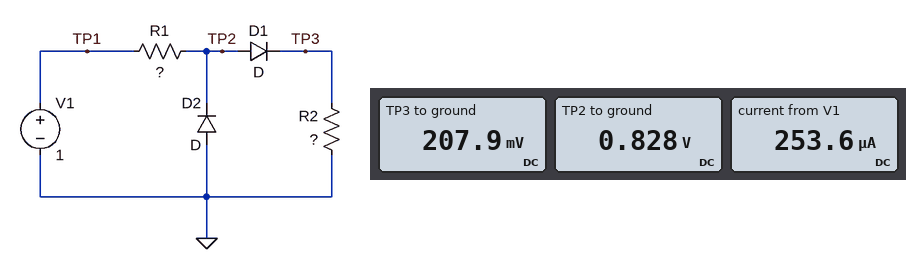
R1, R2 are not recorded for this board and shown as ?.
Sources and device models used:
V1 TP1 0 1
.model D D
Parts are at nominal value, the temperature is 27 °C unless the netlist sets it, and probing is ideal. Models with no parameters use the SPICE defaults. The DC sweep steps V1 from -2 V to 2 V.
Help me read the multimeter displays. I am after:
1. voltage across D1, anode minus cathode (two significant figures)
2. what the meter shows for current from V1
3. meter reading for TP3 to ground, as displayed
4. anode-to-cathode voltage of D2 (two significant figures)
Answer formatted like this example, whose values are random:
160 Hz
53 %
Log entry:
620 mV
253.6 µA
207.9 mV
-830 mV
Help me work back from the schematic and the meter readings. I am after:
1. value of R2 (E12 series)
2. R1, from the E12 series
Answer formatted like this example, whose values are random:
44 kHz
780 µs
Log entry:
820 Ω
680 Ω
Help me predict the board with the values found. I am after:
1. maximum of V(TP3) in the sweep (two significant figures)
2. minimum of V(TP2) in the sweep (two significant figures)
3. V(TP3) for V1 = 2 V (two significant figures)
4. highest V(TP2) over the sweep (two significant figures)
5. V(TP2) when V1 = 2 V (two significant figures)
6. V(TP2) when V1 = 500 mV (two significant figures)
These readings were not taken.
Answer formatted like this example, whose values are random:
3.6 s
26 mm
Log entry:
740 mV
-670 mV
740 mV
1.4 V
1.4 V
500 mV
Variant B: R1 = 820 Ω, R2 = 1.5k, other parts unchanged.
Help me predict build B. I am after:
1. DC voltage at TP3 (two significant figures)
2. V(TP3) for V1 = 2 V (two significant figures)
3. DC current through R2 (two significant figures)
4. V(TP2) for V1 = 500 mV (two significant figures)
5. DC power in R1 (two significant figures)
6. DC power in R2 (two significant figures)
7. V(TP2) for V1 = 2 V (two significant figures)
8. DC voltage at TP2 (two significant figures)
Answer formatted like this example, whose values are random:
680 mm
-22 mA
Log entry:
250 mV
880 mV
170 µA
500 mV
23 µW
43 µW
1.5 V
860 mV
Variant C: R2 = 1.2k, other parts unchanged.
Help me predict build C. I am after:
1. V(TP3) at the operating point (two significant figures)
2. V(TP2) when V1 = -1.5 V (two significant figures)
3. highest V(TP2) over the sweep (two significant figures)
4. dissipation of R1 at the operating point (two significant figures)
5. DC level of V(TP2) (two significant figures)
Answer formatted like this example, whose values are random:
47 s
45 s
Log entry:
250 mV
-660 mV
1.5 V
29 µW
860 mV
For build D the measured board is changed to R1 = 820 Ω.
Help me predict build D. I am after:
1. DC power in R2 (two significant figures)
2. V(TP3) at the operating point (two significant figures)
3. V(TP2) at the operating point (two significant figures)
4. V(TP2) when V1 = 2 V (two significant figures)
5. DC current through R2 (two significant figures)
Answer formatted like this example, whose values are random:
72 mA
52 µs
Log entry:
45 µW
190 mV
810 mV
1.3 V
230 µA
